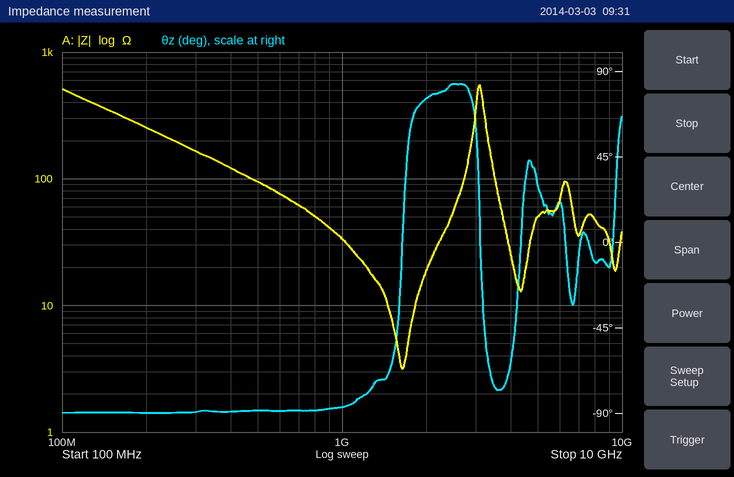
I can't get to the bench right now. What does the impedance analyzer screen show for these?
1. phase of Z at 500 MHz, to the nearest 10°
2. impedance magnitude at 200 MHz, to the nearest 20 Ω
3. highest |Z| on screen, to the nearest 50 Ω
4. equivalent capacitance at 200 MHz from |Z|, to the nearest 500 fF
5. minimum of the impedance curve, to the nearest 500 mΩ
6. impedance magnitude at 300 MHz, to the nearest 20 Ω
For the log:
-90°
260 Ω
550 Ω
3.0 pF
3.0 Ω
160 Ω
